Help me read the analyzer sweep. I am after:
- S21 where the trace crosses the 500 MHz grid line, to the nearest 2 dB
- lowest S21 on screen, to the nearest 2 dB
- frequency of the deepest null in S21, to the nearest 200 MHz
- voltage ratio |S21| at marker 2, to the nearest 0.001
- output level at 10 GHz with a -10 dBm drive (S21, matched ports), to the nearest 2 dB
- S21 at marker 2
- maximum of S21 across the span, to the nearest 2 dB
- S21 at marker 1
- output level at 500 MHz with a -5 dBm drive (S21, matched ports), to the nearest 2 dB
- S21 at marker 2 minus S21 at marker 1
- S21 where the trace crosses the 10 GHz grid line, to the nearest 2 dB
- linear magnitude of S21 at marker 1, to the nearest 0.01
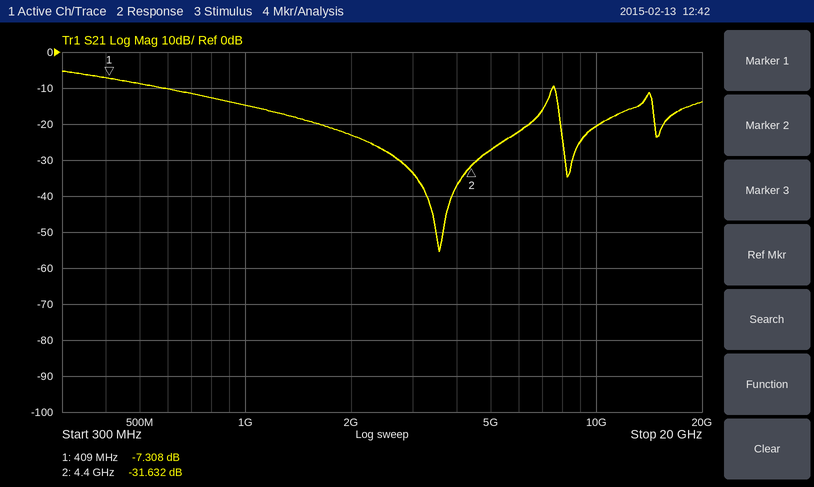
-8 dB
-56 dB
3.6 GHz
0.026
-30 dBm
-31.632 dB
-6 dB
-7.308 dB
-14 dBm
-24.324 dB
-20 dB
0.43
